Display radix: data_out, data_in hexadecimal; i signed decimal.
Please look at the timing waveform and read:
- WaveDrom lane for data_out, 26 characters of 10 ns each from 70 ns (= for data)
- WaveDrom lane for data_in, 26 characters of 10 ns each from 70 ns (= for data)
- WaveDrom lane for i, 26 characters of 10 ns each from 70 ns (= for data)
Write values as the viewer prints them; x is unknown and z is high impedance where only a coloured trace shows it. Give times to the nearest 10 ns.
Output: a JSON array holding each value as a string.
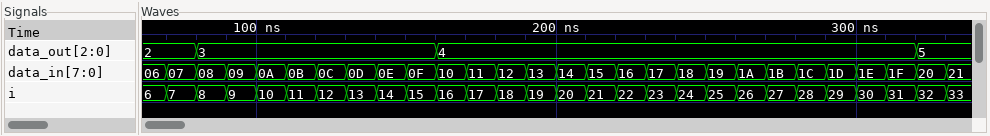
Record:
["{name: 'data_out', wave: '==.......=...............=', data: '2 3 4 5'}", "{name: 'data_in', wave: '==========================', data: '07 08 09 0A 0B 0C 0D 0E 0F 10 11 12 13 14 15 16 17 18 19 1A 1B 1C 1D 1E 1F 20'}", "{name: 'i', wave: '==========================', data: '7 8 9 10 11 12 13 14 15 16 17 18 19 20 21 22 23 24 25 26 27 28 29 30 31 32'}"]
